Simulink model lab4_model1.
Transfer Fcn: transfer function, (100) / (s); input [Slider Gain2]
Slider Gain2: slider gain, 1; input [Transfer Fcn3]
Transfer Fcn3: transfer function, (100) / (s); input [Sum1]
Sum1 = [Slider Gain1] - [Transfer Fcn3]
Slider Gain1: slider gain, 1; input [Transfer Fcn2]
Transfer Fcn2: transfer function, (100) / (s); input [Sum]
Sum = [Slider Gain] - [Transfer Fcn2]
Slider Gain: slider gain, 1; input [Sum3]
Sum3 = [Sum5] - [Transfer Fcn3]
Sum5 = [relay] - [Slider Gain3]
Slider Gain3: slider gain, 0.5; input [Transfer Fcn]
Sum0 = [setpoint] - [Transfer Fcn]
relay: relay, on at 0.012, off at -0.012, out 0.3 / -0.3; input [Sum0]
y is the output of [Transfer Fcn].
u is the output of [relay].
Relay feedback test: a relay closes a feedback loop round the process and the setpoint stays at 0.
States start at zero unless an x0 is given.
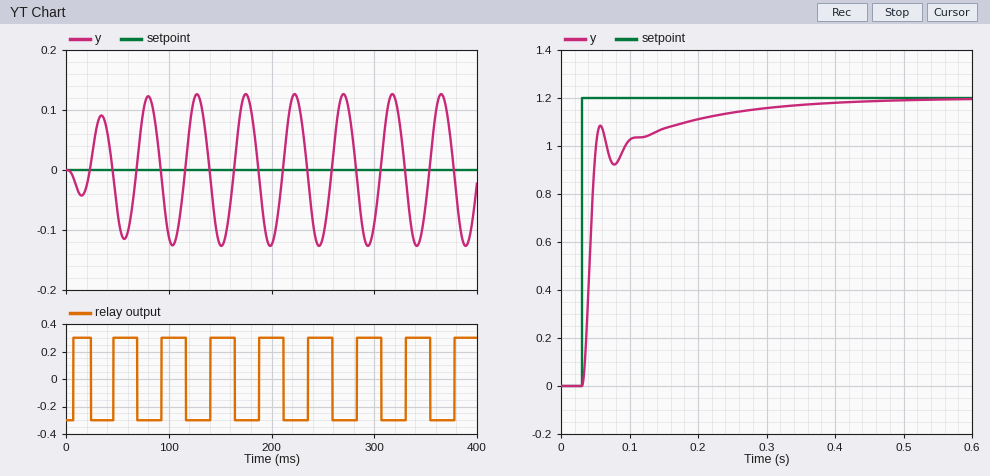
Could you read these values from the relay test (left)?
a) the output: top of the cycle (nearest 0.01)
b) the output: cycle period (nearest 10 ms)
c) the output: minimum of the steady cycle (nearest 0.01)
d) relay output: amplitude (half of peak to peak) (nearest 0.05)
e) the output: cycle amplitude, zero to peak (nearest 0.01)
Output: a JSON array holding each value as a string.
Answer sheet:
["0.13", "50 ms", "-0.13", "0.30", "0.13"]
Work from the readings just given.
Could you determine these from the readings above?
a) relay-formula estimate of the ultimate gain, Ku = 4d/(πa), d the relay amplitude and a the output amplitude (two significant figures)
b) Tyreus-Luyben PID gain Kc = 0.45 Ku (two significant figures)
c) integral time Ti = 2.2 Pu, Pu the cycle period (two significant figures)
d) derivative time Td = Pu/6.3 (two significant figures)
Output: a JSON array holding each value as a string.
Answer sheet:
["2.9", "1.3", "110 ms", "7.9 ms"]
